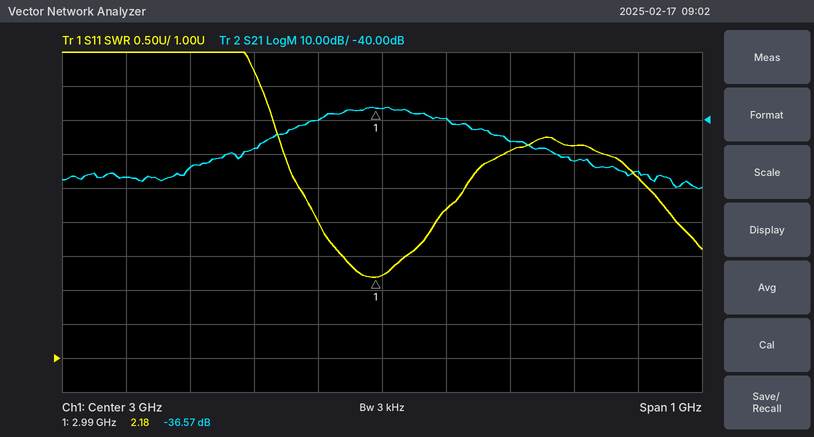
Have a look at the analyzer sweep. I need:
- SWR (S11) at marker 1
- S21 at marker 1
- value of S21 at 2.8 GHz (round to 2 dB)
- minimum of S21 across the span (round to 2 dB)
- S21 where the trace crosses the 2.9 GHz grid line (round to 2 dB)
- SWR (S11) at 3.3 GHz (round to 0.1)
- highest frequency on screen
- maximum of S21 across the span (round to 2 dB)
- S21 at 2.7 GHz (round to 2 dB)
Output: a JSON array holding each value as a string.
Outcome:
["2.18", "-36.57 dB", "-48 dB", "-60 dB", "-40 dB", "4.1", "3.5 GHz", "-36 dB", "-54 dB"]
